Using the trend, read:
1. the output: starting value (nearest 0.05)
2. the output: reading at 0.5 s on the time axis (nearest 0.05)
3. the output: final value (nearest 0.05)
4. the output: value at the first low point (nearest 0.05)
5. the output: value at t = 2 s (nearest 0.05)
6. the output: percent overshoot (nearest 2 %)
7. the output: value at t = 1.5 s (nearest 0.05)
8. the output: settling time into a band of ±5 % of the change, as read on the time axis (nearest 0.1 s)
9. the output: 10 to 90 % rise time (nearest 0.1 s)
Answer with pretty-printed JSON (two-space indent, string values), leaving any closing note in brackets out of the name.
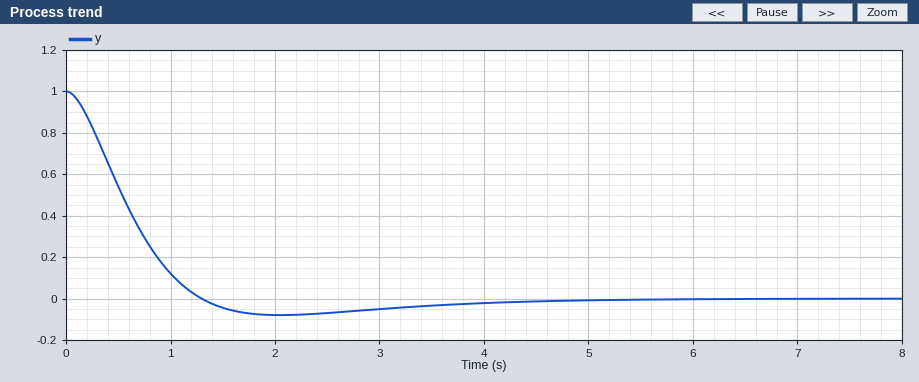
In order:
{
  "the output: starting value": "1.00",
  "the output: reading at 0.5 s on the time axis": "0.55",
  "the output: final value": "0.00",
  "the output: value at the first low point": "-0.10",
  "the output: value at t = 2 s": "-0.10",
  "the output: percent overshoot": "8 %",
  "the output: value at t = 1.5 s": "-0.05",
  "the output: settling time into a band of ±5 % of the change, as read on the time axis": "3.0 s",
  "the output: 10 to 90 % rise time": "0.9 s"
}
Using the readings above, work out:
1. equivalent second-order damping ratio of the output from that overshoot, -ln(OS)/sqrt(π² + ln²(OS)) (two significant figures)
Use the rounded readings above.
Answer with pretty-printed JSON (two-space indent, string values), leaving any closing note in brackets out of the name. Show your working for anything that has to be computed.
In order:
{
  "equivalent second-order damping ratio of the output from that overshoot, -ln(OS)/sqrt(π² + ln²(OS))": "ln(0.08) = -2.526; 2.526 / sqrt(9.870 + 6.379) = 0.63"
}
